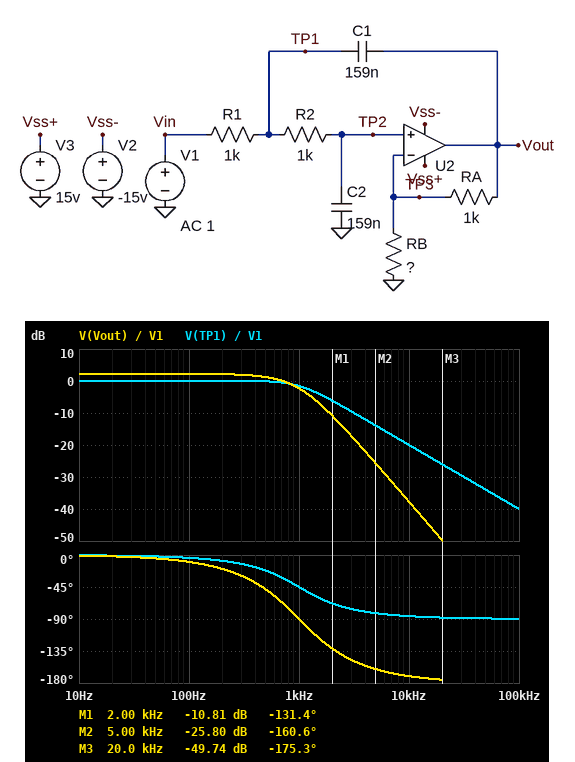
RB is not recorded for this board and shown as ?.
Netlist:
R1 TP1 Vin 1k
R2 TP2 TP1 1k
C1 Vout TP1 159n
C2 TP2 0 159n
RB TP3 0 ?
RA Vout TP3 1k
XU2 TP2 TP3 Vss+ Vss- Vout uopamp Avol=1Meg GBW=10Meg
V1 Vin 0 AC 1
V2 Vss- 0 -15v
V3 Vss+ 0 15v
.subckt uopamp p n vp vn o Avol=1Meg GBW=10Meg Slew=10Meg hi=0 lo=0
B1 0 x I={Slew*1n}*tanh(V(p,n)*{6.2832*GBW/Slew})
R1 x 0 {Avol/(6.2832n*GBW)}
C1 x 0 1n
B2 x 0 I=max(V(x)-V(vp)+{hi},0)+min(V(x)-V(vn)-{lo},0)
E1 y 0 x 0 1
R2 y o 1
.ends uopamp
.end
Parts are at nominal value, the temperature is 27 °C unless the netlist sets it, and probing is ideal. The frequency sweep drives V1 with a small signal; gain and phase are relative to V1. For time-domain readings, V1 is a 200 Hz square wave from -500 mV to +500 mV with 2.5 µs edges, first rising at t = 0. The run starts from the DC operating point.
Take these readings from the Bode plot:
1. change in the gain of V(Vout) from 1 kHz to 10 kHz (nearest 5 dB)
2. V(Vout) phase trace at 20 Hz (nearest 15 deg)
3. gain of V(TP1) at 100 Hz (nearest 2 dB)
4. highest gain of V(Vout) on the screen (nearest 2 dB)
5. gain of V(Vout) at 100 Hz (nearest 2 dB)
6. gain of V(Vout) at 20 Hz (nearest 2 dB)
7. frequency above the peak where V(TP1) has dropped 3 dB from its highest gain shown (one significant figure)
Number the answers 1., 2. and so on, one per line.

1. -35 dB
2. 0 deg
3. 0 dB
4. 2 dB
5. 2 dB
6. 2 dB
7. 1 kHz
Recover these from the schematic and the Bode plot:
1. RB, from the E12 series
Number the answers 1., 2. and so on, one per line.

1. 3.3 kΩ
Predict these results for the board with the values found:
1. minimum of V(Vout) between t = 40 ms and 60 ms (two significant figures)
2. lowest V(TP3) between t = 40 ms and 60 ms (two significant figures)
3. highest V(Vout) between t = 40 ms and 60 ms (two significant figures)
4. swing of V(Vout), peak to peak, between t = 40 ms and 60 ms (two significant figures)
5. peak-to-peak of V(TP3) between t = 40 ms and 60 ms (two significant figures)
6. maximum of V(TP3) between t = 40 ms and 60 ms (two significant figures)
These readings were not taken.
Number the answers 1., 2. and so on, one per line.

1. -660 mV
2. -510 mV
3. 660 mV
4. 1.3 V
5. 1.0 V
6. 510 mV
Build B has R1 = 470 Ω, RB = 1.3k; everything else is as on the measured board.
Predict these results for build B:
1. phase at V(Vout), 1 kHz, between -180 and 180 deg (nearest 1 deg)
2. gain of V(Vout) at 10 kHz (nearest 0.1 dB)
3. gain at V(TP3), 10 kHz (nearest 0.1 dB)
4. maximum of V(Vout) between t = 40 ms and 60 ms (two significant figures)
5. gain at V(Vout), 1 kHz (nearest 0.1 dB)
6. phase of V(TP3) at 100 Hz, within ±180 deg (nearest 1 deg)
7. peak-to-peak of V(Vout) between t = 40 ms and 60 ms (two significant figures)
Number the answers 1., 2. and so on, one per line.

1. -64 deg
2. -28.5 dB
3. -33.5 dB
4. 910 mV
5. 3.2 dB
6. -6 deg
7. 1.8 V
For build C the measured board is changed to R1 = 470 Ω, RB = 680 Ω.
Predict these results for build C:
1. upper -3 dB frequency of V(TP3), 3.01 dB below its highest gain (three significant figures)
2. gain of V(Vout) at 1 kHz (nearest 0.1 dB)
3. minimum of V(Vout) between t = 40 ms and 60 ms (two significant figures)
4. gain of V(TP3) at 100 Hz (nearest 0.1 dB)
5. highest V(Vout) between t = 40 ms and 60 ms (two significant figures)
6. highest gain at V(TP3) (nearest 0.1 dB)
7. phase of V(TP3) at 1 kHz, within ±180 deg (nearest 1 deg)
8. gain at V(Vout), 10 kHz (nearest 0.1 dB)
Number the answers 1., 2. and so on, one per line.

1. 1.66 kHz
2. 8.4 dB
3. -1.5 V
4. 0 dB
5. 1.5 V
6. 0.6 dB
7. -56 deg
8. -25.5 dB
